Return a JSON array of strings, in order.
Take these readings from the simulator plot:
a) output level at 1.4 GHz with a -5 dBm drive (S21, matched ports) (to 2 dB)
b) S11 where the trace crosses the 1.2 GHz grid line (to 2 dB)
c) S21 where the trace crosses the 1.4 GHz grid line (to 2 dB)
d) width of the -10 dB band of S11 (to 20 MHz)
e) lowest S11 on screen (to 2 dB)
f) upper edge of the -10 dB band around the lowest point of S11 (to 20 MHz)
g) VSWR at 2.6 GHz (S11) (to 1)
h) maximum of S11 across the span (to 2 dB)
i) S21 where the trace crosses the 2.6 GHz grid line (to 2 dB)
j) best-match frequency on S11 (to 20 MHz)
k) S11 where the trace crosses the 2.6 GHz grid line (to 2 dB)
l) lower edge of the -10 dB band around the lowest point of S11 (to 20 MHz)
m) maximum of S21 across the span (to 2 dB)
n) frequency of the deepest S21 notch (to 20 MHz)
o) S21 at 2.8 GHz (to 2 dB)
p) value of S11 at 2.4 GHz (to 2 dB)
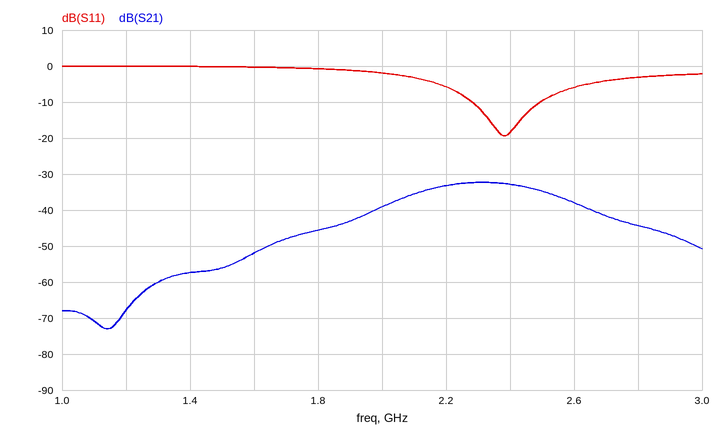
["-62 dBm", "0 dB", "-58 dB", "220 MHz", "-20 dB", "2.50 GHz", "3", "0 dB", "-38 dB", "2.38 GHz", "-6 dB", "2.28 GHz", "-32 dB", "1.14 GHz", "-44 dB", "-18 dB"]
